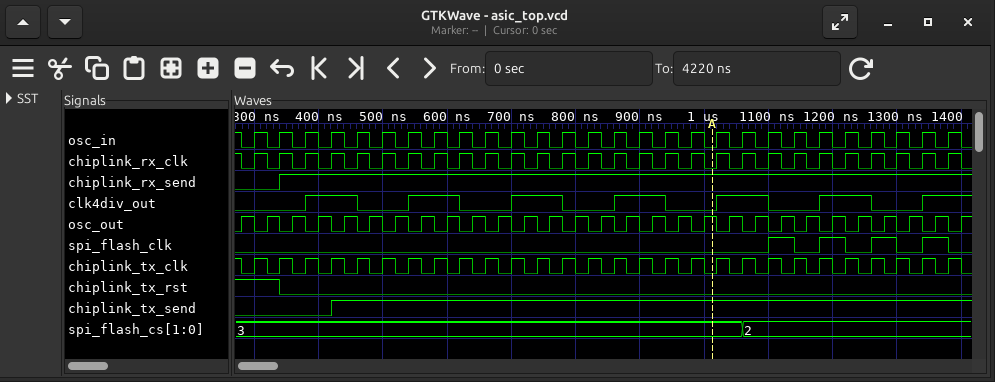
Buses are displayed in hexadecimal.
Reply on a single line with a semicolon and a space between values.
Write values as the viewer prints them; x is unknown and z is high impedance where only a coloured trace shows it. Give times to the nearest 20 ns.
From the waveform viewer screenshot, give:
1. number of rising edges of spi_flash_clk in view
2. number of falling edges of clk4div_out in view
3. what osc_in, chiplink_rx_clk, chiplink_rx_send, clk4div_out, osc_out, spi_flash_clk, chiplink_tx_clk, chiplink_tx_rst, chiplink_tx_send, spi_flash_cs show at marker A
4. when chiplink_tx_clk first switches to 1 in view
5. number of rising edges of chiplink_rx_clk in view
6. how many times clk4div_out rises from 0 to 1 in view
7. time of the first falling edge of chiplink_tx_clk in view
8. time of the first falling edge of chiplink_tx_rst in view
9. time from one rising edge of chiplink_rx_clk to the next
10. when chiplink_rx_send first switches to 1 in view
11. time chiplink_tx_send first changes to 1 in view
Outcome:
4; 6; osc_in=0, chiplink_rx_clk=0, chiplink_rx_send=1, clk4div_out=0, osc_out=1, spi_flash_clk=0, chiplink_tx_clk=0, chiplink_tx_rst=0, chiplink_tx_send=1, spi_flash_cs=3; 300 ns; 28; 7; 280 ns; 340 ns; 40 ns; 340 ns; 420 ns
